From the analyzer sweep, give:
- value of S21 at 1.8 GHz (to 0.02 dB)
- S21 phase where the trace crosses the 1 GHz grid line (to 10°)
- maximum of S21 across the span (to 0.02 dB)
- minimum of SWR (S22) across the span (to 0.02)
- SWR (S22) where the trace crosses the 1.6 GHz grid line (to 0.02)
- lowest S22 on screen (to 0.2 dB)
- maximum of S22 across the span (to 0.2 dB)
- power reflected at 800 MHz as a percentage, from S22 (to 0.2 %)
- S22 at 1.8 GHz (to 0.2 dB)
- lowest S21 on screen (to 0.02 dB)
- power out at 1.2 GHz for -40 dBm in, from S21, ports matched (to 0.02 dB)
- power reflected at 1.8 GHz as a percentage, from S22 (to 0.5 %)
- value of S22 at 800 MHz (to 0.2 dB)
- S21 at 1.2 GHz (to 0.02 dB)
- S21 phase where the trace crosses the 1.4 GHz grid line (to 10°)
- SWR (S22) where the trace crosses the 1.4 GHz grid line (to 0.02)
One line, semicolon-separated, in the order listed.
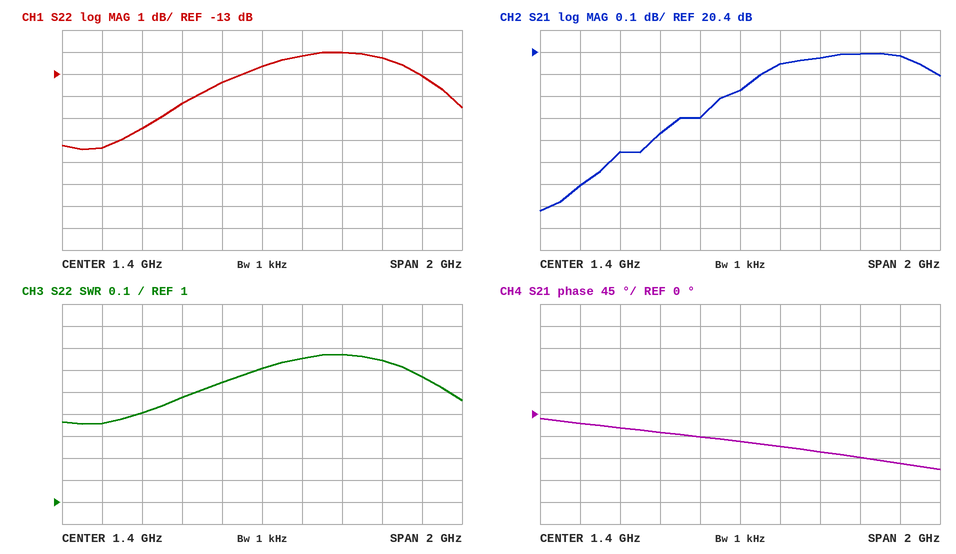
20.38 dB; -40°; 20.40 dB; 1.36; 1.66; -16.4 dB; -12.0 dB; 2.8 %; -12.0 dB; 19.68 dB; -19.90 dBm; 6.5 %; -15.4 dB; 20.10 dB; -60°; 1.60
